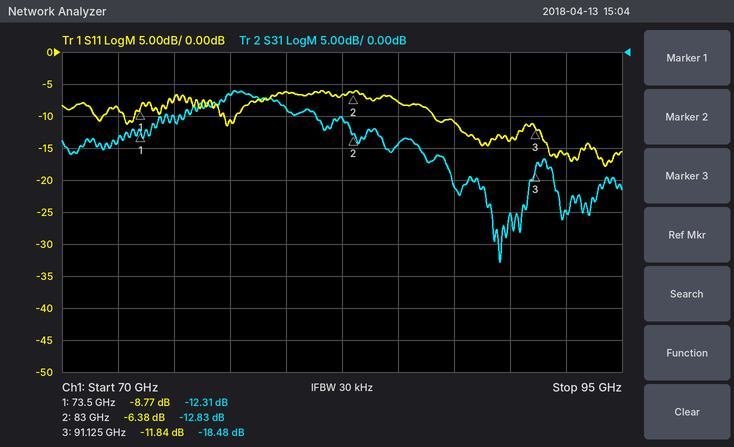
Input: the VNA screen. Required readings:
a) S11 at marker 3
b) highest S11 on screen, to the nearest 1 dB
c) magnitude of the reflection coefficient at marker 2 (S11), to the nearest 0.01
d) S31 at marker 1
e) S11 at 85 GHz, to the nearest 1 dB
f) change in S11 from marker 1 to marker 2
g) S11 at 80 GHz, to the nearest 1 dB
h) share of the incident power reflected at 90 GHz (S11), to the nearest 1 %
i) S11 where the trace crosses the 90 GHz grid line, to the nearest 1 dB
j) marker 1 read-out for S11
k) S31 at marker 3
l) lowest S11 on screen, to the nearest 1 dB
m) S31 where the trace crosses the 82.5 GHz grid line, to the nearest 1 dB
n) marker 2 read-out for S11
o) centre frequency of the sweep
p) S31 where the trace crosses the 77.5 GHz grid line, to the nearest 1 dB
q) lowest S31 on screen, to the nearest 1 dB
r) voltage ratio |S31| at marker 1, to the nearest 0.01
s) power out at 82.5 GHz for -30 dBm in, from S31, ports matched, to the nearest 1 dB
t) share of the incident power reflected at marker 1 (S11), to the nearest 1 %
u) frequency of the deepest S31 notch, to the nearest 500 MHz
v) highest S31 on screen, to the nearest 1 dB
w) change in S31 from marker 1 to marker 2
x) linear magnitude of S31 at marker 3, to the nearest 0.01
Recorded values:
-11.84 dB
-6 dB
0.48
-12.31 dB
-8 dB
2.39 dB
-6 dB
4 %
-14 dB
-8.77 dB
-18.48 dB
-18 dB
-10 dB
-6.38 dB
82.5 GHz
-7 dB
-33 dB
0.24
-40 dBm
13 %
89.5 GHz
-6 dB
-0.52 dB
0.12
